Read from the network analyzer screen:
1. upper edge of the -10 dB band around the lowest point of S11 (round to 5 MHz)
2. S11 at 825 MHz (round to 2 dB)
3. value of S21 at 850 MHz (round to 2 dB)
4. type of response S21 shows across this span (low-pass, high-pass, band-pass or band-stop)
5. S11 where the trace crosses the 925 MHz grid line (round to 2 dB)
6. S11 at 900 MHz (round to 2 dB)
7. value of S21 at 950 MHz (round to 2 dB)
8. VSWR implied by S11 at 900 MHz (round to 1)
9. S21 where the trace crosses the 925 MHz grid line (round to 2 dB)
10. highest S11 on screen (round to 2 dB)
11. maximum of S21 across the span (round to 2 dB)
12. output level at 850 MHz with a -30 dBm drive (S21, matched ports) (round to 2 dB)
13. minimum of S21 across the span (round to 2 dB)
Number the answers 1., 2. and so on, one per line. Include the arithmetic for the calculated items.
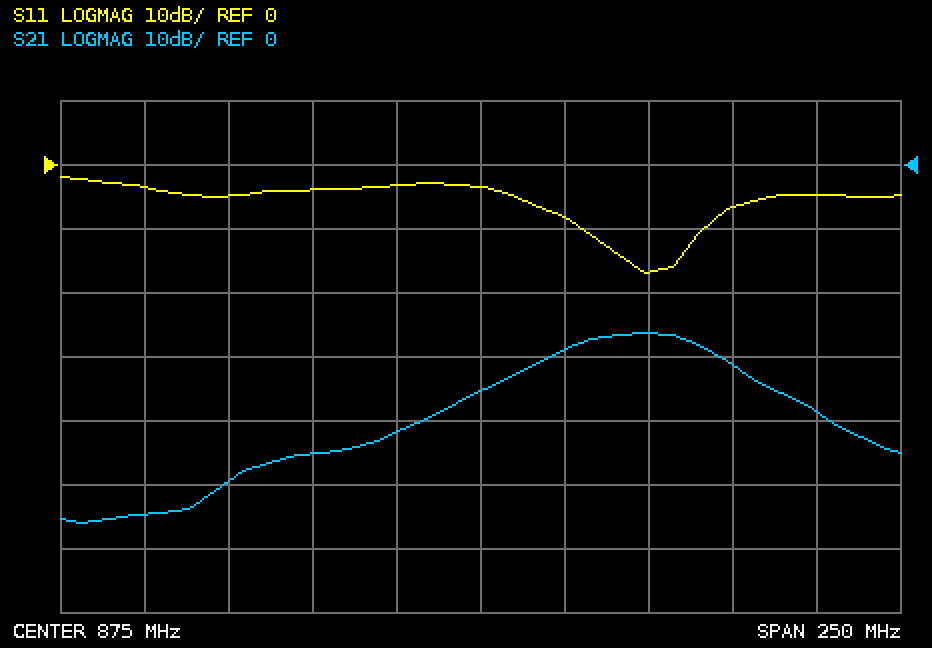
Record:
1. 940 MHz
2. -4 dB
3. -42 dB
4. band-pass
5. -16 dB
6. -8 dB
7. -32 dB
8. |Γ| = 10^(-8/20) = 0.3981; VSWR = (1 + 0.3981)/(1 − 0.3981) ≈ 2
9. -26 dB
10. -2 dB
11. -26 dB
12. -30 dBm + (-42 dB) = -72 dBm
13. -56 dB
